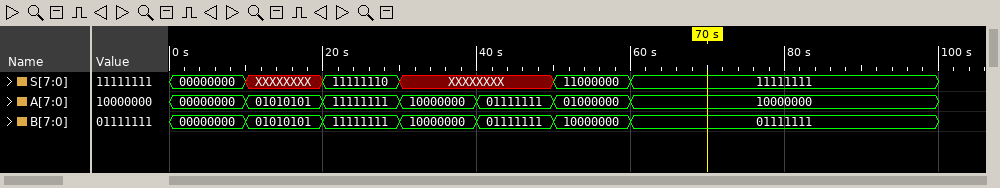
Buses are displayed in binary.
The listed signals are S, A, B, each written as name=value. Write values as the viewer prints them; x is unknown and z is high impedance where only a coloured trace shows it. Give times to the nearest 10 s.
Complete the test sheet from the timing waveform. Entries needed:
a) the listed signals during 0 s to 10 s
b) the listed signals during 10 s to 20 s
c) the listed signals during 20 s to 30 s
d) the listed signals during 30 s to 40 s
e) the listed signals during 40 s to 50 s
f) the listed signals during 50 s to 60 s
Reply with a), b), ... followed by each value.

a) S=00000000, A=00000000, B=00000000
b) S=XXXXXXXX, A=01010101, B=01010101
c) S=11111110, A=11111111, B=11111111
d) S=XXXXXXXX, A=10000000, B=10000000
e) S=XXXXXXXX, A=01111111, B=01111111
f) S=11000000, A=01000000, B=10000000
